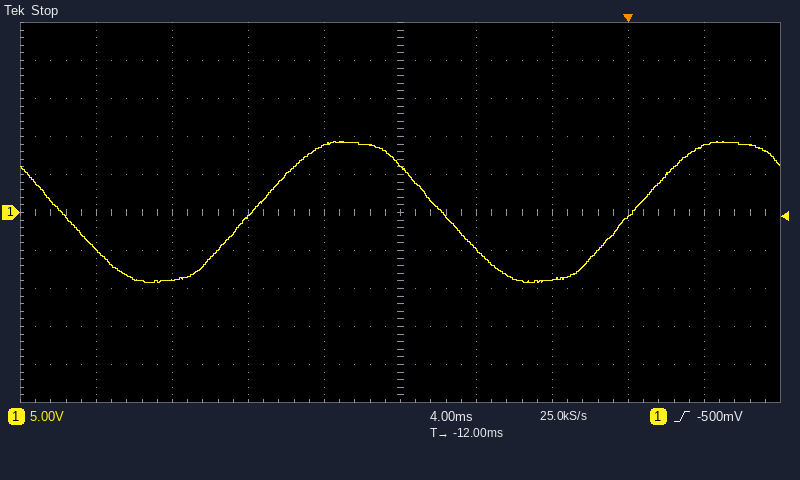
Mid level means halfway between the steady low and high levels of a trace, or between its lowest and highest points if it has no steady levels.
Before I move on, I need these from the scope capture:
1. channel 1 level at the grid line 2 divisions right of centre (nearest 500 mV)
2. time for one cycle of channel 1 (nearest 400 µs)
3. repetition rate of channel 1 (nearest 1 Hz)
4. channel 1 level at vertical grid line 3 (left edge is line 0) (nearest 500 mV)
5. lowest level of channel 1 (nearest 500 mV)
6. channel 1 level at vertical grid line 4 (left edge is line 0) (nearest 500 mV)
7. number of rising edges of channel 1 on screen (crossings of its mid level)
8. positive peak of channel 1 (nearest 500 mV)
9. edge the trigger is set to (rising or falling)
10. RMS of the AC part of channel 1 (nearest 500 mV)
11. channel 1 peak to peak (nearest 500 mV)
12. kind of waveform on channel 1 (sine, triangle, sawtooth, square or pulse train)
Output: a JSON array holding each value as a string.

["-9.0 V", "20.0 ms", "50 Hz", "-500 mV", "-9.0 V", "9.0 V", "2", "9.5 V", "rising", "6.5 V", "18.5 V", "sine"]
